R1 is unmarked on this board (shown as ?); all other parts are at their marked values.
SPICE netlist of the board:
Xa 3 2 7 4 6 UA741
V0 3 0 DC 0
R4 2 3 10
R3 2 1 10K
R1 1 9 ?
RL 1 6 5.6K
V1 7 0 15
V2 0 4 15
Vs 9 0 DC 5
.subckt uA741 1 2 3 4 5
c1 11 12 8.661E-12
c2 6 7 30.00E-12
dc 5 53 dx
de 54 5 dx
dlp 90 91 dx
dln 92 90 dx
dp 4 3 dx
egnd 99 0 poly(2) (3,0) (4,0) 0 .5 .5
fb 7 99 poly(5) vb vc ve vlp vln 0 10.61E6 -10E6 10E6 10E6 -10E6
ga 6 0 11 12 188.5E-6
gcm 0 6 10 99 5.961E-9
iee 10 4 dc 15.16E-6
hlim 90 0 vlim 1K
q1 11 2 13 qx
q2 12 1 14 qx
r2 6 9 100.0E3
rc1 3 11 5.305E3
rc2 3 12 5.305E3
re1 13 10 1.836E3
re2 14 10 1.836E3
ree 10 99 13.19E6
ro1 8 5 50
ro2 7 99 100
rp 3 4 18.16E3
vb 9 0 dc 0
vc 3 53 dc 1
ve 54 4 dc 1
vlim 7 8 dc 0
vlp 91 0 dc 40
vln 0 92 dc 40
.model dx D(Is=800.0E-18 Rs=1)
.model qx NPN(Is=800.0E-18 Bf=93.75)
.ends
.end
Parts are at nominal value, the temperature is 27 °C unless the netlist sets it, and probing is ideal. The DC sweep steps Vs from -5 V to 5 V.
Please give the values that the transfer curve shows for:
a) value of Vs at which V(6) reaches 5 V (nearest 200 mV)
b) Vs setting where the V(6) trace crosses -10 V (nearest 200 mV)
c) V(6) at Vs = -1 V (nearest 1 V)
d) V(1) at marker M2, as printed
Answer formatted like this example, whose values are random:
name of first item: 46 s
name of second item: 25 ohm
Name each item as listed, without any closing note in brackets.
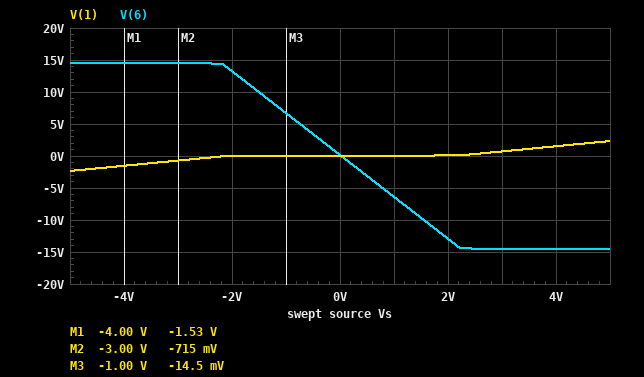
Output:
value of Vs at which V(6) reaches 5 V: -800 mV
Vs setting where the V(6) trace crosses -10 V: 1.6 V
V(6) at Vs = -1 V: 7 V
V(1) at marker M2, as printed: -715 mV
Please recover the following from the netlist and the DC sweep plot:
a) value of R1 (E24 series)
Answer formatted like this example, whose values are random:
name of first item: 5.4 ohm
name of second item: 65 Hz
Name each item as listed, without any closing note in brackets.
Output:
value of R1: 820 Ω
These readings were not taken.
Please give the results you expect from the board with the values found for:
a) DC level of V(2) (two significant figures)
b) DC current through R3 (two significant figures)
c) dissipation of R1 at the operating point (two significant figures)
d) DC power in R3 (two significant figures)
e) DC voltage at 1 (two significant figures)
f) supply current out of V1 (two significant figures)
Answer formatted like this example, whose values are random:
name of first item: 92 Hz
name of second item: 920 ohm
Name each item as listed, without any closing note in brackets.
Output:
DC level of V(2): 2.3 mV
DC current through R3: 230 µA
dissipation of R1 at the operating point: 8.6 mW
DC power in R3: 550 µW
DC voltage at 1: 2.3 V
supply current out of V1: 1.7 mA
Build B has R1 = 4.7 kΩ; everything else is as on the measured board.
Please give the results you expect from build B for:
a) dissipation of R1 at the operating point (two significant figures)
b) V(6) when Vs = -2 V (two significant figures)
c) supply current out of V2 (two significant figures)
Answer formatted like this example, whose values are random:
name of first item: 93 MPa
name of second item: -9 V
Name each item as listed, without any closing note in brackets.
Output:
dissipation of R1 at the operating point: 5.2 mW
V(6) when Vs = -2 V: 2.4 V
supply current out of V2: 1.7 mA
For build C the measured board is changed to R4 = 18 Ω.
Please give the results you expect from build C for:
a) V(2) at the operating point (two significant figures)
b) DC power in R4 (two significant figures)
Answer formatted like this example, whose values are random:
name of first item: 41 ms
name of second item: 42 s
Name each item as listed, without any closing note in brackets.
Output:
V(2) at the operating point: 4.2 mV
DC power in R4: 980 nW
